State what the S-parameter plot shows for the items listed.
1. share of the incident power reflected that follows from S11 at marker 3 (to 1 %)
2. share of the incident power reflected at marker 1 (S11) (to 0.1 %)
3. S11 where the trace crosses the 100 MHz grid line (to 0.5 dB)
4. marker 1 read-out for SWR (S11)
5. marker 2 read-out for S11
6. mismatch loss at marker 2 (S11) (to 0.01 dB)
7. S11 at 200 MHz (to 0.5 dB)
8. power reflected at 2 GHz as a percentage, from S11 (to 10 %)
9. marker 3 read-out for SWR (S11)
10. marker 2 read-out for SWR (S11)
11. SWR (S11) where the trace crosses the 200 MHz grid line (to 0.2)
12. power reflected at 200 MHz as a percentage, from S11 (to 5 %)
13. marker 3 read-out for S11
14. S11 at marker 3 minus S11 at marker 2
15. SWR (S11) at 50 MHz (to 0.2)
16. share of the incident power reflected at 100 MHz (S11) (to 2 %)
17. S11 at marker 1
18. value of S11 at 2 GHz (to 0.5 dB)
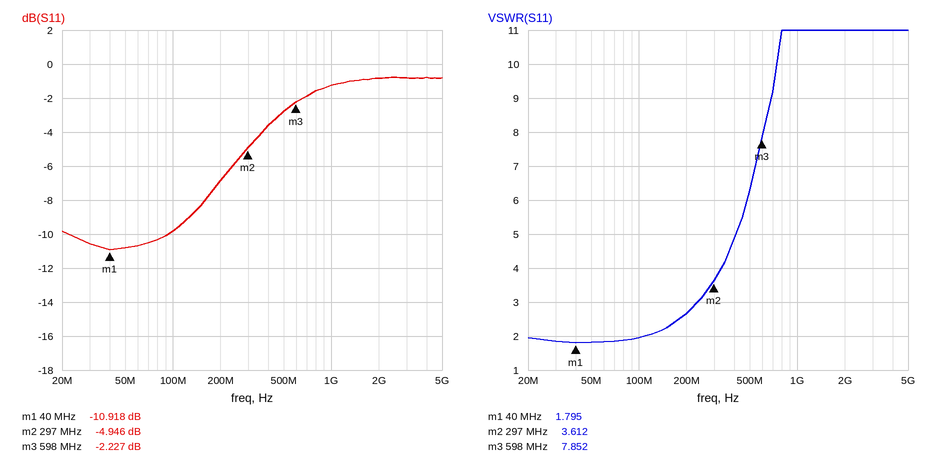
60 %
8.1 %
-10.0 dB
1.795
-4.946 dB
1.68 dB
-7.0 dB
80 %
7.852
3.612
2.6
20 %
-2.227 dB
2.719 dB
1.8
10 %
-10.918 dB
-1.0 dB
